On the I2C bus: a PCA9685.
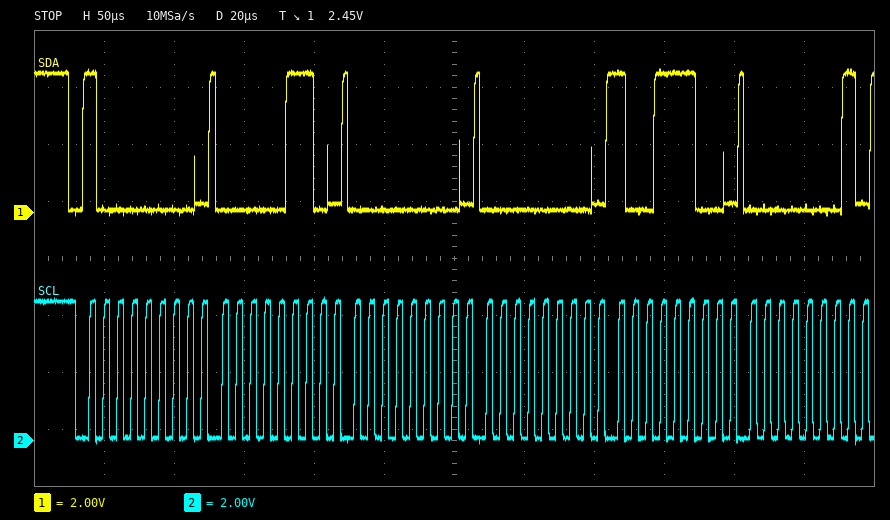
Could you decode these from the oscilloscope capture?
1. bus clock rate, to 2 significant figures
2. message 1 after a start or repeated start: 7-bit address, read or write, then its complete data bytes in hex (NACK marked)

100 kHz
0x40 write: 06 00 00 9C 01
